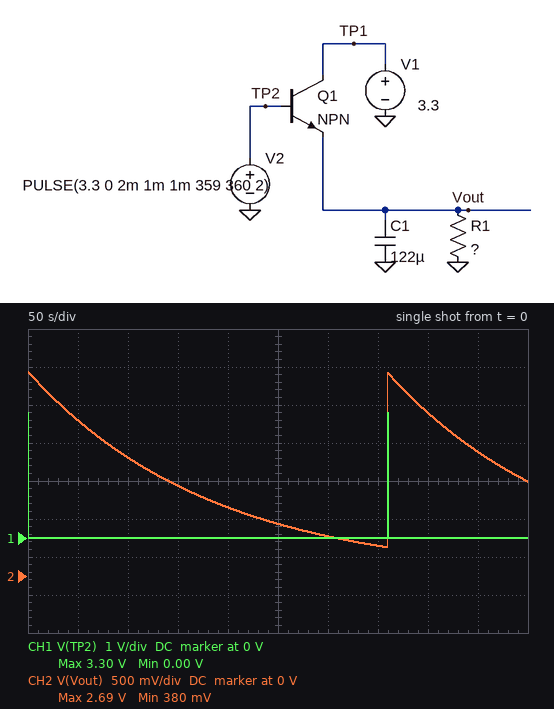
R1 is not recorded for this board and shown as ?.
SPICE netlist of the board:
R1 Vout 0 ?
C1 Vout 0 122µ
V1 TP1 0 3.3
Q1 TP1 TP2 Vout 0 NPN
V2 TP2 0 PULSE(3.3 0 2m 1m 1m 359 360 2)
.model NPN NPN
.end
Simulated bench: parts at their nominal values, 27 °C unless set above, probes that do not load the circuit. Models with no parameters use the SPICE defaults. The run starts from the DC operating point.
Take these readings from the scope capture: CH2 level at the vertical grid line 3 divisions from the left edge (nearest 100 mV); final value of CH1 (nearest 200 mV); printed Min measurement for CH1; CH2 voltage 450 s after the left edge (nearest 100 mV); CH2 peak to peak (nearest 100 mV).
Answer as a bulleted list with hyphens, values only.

- 1.2 V
- 0 V
- 0.00 V
- 1.6 V
- 2.3 V
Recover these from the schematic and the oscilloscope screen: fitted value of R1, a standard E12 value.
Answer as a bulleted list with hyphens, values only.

- 1.5 MΩ
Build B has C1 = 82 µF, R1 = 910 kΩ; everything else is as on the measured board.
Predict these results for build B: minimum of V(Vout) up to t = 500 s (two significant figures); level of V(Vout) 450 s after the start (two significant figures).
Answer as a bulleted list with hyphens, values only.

- 22 mV
- 800 mV
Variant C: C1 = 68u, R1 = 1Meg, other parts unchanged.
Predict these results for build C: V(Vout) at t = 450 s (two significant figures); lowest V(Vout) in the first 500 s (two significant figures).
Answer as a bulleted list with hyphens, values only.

- 710 mV
- 14 mV
